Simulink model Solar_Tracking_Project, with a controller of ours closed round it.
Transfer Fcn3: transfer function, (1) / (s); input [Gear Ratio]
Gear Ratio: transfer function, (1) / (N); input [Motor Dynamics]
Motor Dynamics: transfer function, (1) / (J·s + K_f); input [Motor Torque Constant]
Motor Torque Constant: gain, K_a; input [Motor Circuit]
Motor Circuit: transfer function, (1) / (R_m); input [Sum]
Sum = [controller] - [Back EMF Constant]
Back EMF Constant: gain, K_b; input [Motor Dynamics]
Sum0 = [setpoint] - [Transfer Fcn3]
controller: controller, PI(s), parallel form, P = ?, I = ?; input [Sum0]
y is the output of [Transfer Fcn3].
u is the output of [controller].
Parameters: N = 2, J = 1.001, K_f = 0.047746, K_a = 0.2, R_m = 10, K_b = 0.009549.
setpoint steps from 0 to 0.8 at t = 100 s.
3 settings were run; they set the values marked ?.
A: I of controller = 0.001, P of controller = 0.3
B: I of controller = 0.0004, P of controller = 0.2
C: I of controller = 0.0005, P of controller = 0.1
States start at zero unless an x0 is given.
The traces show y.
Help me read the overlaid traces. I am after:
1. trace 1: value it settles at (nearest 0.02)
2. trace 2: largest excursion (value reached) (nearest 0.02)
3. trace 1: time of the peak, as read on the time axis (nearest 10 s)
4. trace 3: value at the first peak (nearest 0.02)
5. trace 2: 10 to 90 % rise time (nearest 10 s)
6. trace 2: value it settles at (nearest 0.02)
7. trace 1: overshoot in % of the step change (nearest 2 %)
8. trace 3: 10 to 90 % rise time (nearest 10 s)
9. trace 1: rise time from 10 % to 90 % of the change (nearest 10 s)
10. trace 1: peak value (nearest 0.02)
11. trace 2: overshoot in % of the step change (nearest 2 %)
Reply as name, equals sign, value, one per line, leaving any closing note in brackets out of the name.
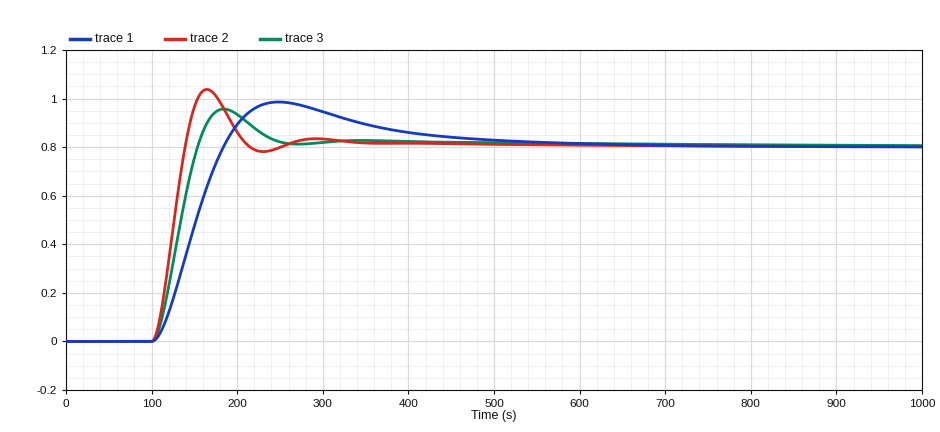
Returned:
trace 1: value it settles at = 0.80
trace 2: largest excursion (value reached) = 1.04
trace 1: time of the peak, as read on the time axis = 250 s
trace 3: value at the first peak = 0.96
trace 2: 10 to 90 % rise time = 30 s
trace 2: value it settles at = 0.80
trace 1: overshoot in % of the step change = 24 %
trace 3: 10 to 90 % rise time = 40 s
trace 1: rise time from 10 % to 90 % of the change = 60 s
trace 1: peak value = 0.98
trace 2: overshoot in % of the step change = 30 %
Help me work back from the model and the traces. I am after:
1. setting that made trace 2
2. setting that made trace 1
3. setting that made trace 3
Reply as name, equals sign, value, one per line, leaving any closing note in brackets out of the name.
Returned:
setting that made trace 2 = A
setting that made trace 1 = C
setting that made trace 3 = B
